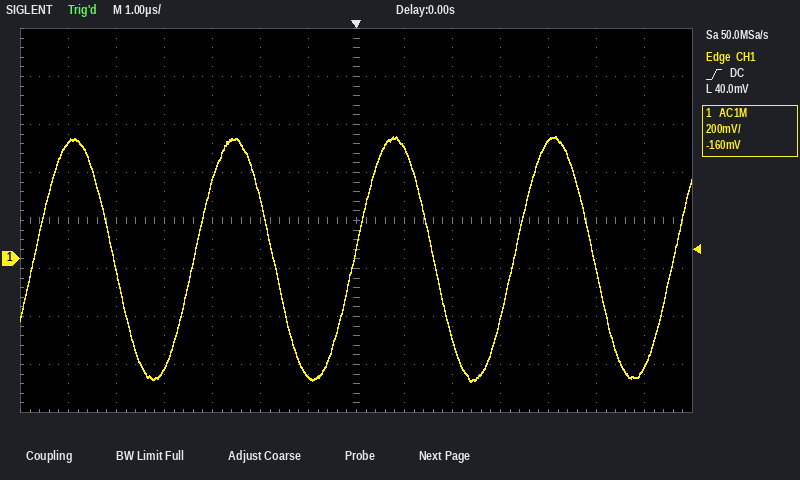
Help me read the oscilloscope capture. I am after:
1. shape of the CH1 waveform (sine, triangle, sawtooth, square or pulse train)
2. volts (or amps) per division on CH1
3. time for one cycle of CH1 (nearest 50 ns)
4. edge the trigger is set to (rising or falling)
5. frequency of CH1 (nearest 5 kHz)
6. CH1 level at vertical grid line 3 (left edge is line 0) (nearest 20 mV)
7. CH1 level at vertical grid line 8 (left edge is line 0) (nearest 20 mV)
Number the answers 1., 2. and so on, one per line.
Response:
1. sine
2. 200 mV
3. 3.35 µs
4. rising
5. 300 kHz
6. -460 mV
7. 460 mV
